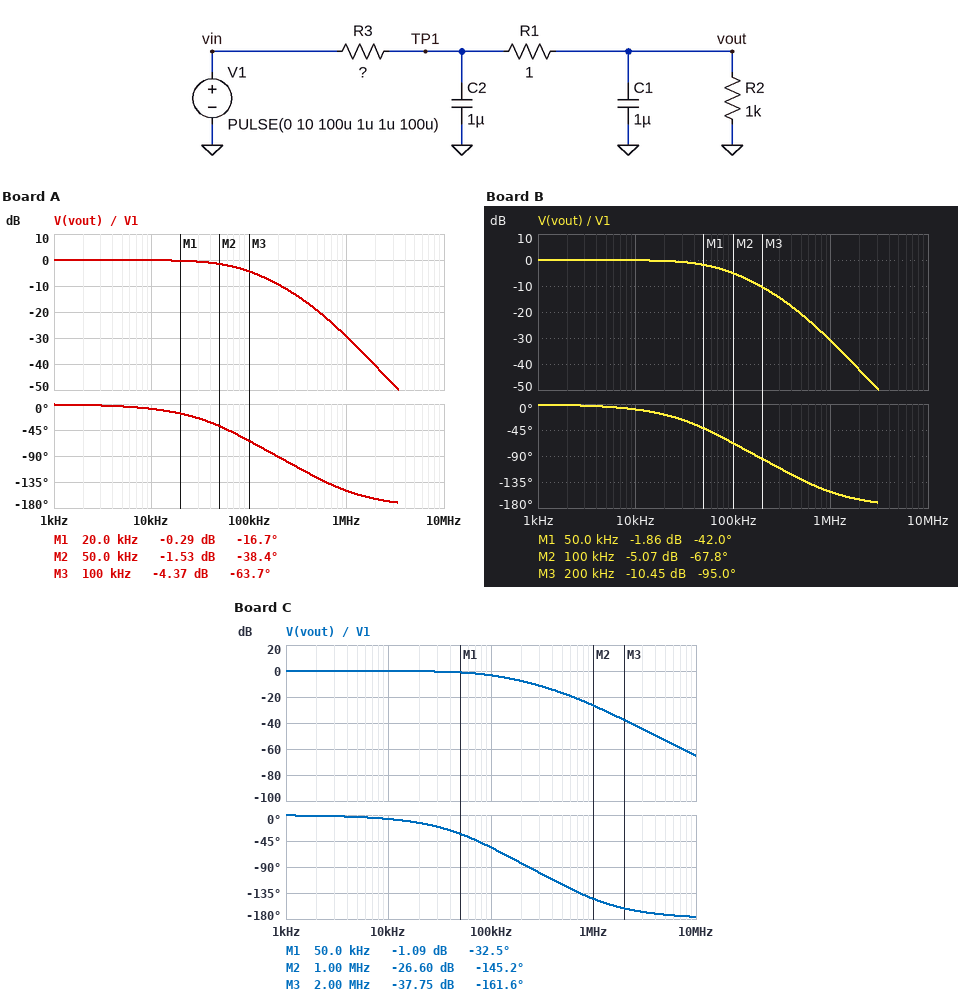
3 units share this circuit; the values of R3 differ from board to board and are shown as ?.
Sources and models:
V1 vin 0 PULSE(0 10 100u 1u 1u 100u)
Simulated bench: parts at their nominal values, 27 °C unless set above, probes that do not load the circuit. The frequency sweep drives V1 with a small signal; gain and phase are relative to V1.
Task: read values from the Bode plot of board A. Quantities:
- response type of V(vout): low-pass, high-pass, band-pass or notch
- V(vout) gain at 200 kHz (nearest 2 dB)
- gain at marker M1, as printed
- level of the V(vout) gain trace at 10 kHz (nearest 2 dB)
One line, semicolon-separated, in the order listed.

low-pass; -10 dB; -0.29 dB; 0 dB
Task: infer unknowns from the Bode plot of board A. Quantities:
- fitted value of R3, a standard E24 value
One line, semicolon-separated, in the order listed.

0.68 Ω
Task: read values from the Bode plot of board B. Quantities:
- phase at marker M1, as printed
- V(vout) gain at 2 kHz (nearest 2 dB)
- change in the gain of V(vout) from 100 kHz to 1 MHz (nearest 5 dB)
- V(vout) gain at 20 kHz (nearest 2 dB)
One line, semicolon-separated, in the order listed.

-42.0 deg; 0 dB; -25 dB; 0 dB
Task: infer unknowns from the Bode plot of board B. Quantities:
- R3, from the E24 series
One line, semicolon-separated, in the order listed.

0.82 Ω
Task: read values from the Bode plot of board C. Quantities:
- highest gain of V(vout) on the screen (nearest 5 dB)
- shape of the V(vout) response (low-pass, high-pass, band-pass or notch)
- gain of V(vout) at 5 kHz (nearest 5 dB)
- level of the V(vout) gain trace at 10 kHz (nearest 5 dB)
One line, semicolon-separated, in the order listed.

0 dB; low-pass; 0 dB; 0 dB
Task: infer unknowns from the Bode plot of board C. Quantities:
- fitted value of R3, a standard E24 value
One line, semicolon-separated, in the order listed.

0.47 Ω
